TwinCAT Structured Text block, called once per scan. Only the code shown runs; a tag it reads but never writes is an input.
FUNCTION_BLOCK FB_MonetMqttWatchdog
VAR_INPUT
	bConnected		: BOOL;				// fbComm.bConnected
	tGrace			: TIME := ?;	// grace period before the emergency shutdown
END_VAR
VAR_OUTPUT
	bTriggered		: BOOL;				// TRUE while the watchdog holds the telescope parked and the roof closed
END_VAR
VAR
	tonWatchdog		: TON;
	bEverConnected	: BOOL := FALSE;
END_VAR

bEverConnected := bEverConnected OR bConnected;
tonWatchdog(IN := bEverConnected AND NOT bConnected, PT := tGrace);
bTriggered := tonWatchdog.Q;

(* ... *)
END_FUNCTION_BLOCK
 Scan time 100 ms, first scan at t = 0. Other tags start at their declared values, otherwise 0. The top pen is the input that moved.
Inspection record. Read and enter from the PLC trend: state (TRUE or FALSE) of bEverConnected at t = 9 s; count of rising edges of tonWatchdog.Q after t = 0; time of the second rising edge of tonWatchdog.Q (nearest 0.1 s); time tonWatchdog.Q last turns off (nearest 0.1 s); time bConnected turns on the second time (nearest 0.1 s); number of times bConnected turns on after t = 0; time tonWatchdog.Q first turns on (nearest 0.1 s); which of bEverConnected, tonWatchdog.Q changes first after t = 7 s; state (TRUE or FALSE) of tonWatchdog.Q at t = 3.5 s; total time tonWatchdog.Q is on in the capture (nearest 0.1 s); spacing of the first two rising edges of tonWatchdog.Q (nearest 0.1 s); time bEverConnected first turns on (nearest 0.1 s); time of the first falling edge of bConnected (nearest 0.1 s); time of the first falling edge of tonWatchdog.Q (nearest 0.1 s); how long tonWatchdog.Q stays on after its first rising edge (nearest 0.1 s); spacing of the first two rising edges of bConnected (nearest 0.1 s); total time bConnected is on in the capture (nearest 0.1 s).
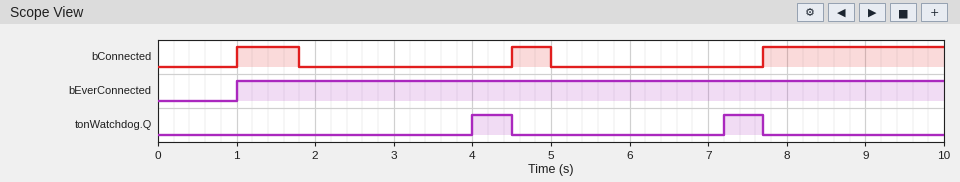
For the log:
TRUE
2
7.2 s
7.7 s
4.5 s
3
4.0 s
tonWatchdog.Q
FALSE
1.0 s
3.2 s
1.0 s
1.8 s
4.5 s
0.5 s
3.5 s
3.6 s
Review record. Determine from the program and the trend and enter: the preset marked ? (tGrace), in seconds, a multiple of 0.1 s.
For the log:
2.2 s
